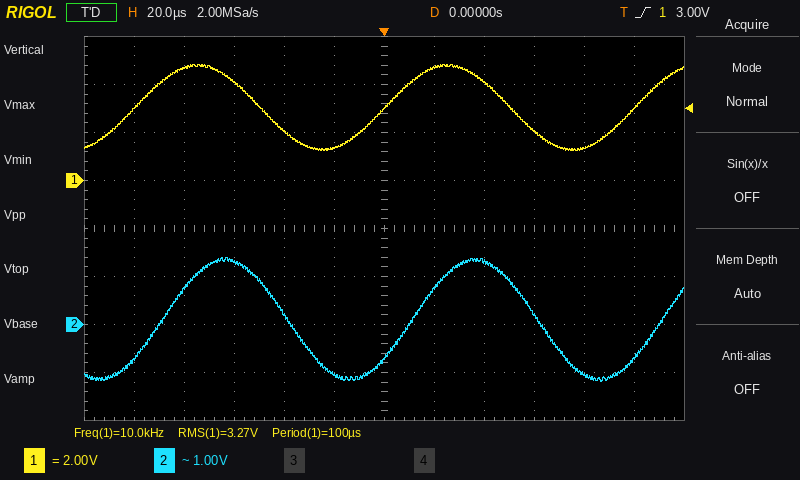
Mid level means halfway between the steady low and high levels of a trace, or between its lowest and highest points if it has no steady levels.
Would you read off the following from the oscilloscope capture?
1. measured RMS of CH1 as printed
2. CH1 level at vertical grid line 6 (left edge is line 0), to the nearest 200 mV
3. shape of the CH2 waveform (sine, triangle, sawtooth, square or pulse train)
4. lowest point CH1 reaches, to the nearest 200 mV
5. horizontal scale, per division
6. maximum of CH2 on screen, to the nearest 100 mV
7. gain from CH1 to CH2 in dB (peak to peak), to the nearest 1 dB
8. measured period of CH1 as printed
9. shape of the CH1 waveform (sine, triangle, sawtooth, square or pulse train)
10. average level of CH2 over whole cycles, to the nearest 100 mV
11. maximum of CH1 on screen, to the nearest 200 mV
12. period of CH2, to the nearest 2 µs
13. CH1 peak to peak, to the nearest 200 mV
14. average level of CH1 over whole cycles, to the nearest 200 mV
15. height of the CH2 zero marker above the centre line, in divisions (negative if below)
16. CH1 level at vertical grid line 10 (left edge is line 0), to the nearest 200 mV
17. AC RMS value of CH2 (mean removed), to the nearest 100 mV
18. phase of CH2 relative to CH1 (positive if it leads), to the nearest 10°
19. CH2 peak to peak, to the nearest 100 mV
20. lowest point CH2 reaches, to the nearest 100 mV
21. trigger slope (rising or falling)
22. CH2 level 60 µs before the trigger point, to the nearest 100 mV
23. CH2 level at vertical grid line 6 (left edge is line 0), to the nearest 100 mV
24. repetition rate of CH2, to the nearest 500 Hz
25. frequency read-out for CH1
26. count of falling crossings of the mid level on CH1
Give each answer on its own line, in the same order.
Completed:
3.27 V
3.0 V
sine
1.2 V
20 µs
1.4 V
-3 dB
100 µs
sine
100 mV
4.8 V
100 µs
3.6 V
3.0 V
-2.0 div
1.4 V
900 mV
-40°
2.6 V
-1.2 V
rising
1.3 V
-700 mV
10.0 kHz
10.0 kHz
2
